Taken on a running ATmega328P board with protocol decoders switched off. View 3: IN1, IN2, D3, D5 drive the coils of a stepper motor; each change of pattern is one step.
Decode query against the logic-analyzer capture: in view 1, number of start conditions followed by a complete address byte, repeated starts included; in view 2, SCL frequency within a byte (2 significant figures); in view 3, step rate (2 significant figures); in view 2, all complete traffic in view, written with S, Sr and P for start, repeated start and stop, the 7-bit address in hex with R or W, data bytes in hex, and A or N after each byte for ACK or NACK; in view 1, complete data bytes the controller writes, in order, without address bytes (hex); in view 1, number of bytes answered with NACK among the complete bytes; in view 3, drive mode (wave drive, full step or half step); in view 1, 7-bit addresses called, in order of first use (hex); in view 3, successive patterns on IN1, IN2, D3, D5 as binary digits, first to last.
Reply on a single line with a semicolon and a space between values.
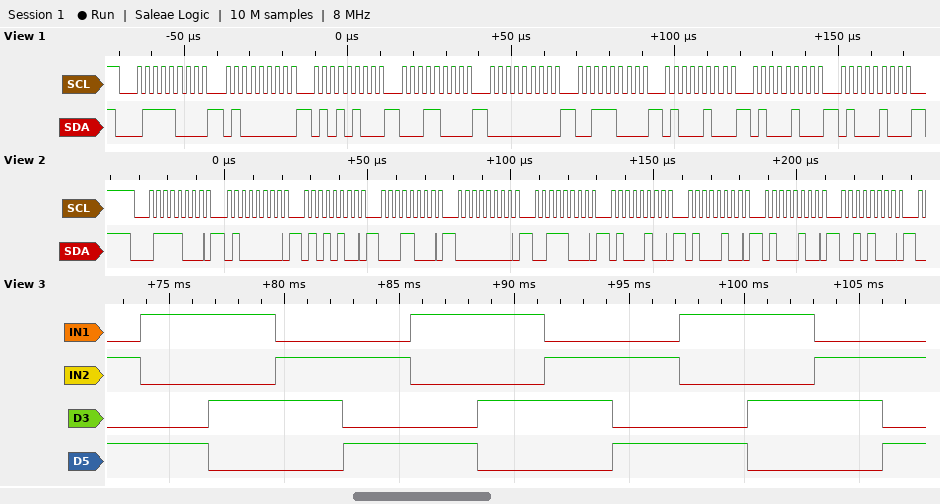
1; 400 kHz; 340 steps/s; S 3CW A 40 A 54 A 18 A 00 A 38 A 44 A 44 A 44 A 28 A; 40 54 18 00 38 44 44 44; 0; full step; 0x3C; 0101 1001 1010 0110 0101 1001 1010 0110 0101 1001 1010 0110 0101
